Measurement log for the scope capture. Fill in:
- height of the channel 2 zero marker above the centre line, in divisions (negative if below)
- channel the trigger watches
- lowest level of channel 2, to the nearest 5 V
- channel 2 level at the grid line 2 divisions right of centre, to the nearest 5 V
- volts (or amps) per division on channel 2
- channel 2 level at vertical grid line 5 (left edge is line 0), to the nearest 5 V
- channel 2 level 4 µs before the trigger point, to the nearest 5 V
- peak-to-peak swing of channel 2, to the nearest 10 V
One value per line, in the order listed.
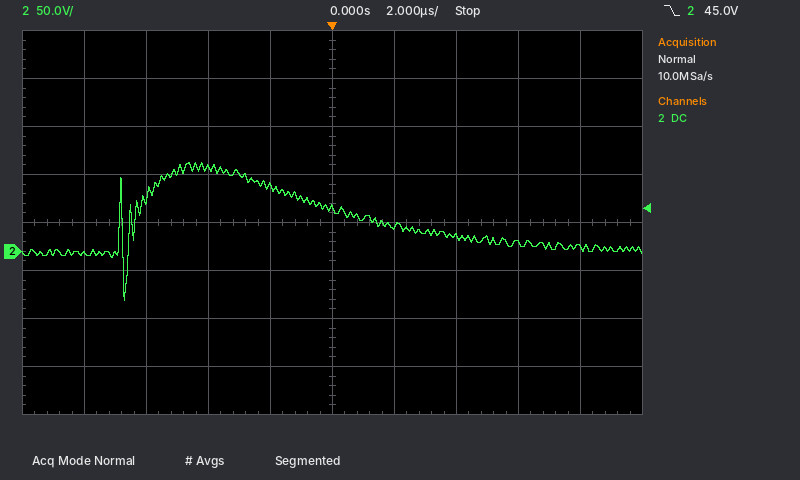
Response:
-0.6 div
channel 2
-50 V
15 V
50 V
45 V
85 V
140 V
